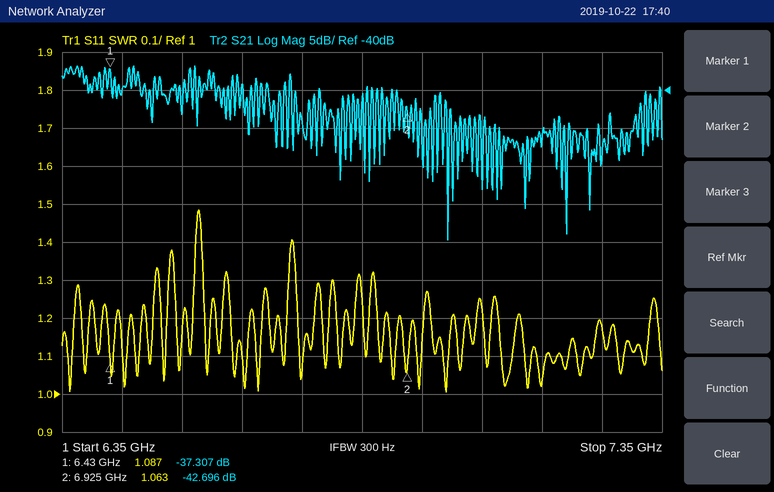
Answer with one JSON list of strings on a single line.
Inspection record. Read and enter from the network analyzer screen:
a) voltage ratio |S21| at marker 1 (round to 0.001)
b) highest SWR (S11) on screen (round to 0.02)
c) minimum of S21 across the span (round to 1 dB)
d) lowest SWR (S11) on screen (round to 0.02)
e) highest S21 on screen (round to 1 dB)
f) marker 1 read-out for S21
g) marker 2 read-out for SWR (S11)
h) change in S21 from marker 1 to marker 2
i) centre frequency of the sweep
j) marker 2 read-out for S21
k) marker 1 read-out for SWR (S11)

["0.014", "1.48", "-60 dB", "1.00", "-37 dB", "-37.307 dB", "1.063", "-5.389 dB", "6.85 GHz", "-42.696 dB", "1.087"]
